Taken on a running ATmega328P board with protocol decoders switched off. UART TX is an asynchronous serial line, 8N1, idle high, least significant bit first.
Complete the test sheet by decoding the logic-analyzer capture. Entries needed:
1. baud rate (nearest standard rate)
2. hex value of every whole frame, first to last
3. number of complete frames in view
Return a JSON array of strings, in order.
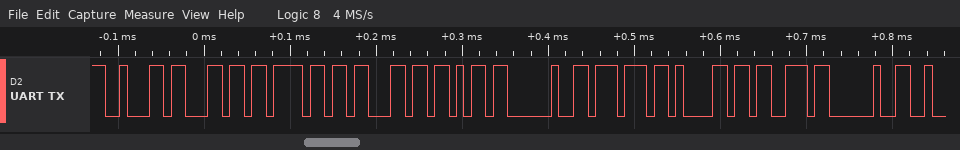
["115200 baud", "0x62 0x6C 0x6F 0x63 0x6B 0x20 0x77 0x61 0x73 0x20", "10"]
